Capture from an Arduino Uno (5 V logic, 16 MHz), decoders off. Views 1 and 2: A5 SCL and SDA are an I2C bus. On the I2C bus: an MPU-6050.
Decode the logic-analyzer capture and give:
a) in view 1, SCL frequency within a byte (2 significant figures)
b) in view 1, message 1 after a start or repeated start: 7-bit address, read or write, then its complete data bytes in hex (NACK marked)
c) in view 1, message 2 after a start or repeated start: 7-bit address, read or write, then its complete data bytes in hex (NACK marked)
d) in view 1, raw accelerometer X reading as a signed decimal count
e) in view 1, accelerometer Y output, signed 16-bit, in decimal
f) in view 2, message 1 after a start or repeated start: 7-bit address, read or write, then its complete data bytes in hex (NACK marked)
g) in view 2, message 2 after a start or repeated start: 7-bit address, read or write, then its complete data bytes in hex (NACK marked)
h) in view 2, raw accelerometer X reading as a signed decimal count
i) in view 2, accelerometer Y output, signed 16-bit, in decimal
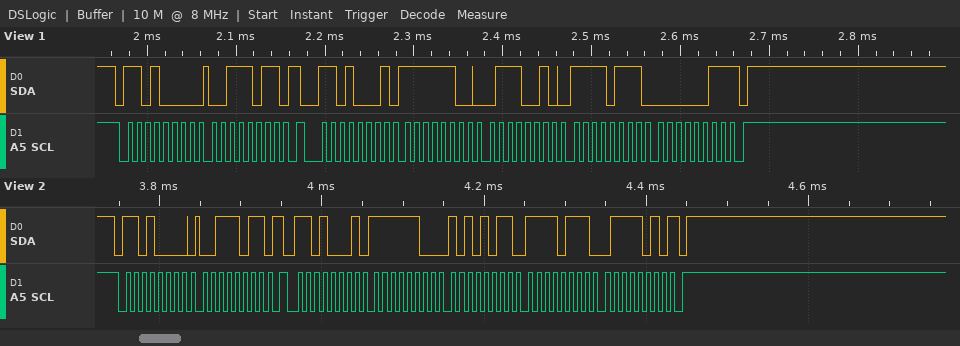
100 kHz
0x68 write: 3B
0x68 read: FC 72 F7 03 NACK
-910
-2301
0x68 write: 3B
0x68 read: FC AB F7 7A NACK
-853
-2182
